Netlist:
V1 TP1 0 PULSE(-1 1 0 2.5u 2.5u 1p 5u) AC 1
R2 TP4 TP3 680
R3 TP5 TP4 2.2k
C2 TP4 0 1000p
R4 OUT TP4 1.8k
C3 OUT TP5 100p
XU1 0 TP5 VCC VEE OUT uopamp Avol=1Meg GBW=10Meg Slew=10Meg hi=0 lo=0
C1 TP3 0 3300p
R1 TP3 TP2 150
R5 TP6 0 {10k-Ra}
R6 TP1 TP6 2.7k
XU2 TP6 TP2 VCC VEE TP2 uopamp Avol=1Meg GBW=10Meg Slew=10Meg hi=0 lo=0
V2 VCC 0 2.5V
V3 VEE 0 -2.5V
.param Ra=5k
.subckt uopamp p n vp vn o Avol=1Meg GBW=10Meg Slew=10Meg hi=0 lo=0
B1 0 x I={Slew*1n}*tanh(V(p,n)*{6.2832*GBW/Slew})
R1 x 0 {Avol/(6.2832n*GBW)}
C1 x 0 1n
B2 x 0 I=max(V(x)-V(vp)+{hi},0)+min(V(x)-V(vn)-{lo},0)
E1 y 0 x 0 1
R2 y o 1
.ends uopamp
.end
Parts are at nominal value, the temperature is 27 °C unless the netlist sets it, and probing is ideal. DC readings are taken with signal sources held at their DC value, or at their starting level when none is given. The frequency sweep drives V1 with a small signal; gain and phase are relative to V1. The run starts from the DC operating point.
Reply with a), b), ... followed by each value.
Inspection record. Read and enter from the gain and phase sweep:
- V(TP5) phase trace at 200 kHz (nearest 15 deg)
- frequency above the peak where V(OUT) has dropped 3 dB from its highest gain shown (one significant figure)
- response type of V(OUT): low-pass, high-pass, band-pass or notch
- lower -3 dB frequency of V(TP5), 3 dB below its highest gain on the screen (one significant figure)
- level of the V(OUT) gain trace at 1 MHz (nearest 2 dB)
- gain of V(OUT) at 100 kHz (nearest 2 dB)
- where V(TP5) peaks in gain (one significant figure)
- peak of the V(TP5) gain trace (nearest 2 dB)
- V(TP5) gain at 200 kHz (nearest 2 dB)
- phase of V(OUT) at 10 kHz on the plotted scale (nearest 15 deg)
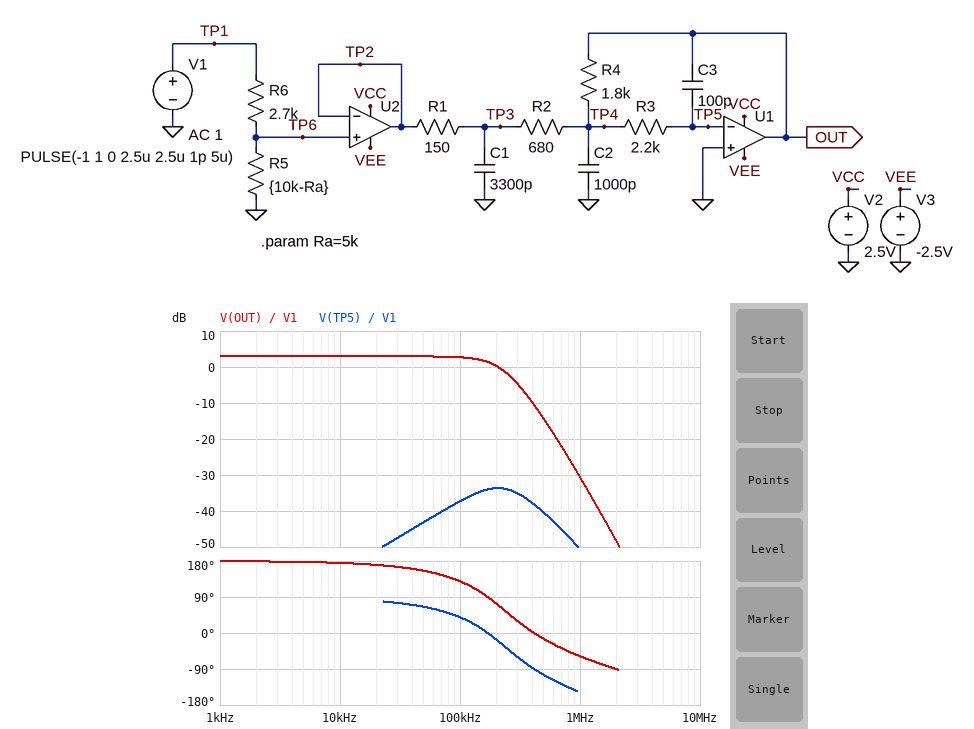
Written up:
a) -15 deg
b) 200 kHz
c) low-pass
d) 100 kHz
e) -30 dB
f) 2 dB
g) 200 kHz
h) -34 dB
i) -34 dB
j) 180 deg
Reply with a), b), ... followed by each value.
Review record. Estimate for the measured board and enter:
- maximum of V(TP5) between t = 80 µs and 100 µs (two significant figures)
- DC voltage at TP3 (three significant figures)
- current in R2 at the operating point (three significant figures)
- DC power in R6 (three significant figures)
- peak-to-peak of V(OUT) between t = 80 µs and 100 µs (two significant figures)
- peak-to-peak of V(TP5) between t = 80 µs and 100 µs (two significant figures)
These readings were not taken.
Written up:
a) 17 mV
b) -532 mV
c) 782 µA
d) 45.5 µW
e) 1.7 V
f) 35 mV
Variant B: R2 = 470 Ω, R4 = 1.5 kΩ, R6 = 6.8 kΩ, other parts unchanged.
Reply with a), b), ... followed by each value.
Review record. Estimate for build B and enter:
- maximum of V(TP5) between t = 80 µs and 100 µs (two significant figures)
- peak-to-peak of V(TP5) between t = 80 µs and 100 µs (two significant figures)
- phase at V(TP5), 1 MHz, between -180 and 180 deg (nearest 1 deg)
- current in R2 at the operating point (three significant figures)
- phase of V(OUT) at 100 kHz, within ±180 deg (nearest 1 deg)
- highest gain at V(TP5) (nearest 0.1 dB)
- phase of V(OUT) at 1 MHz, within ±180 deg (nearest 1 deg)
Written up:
a) 12 mV
b) 24 mV
c) -141 deg
d) 683 µA
e) 130 deg
f) -36.7 dB
g) -51 deg
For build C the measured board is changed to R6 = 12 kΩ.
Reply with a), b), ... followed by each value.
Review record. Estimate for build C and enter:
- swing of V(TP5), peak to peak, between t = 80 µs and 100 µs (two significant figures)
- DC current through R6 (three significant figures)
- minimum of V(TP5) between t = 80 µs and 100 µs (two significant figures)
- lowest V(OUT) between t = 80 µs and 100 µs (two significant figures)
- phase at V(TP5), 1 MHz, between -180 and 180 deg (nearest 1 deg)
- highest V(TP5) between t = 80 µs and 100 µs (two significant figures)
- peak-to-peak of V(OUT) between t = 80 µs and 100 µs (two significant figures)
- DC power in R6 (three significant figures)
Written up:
a) 16 mV
b) 58.8 µA
c) -7.8 mV
d) -380 mV
e) -148 deg
f) 7.8 mV
g) 760 mV
h) 41.5 µW
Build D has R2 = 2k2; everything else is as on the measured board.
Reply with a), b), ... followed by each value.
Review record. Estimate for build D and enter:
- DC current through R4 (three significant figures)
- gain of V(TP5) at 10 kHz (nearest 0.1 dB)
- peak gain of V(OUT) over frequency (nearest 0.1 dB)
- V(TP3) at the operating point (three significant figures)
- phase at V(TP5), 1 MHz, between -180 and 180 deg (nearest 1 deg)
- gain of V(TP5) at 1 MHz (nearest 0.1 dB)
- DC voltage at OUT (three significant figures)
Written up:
a) 276 µA
b) -66.1 dB
c) -5.1 dB
d) -608 mV
e) -159 deg
f) -60.1 dB
g) 497 mV
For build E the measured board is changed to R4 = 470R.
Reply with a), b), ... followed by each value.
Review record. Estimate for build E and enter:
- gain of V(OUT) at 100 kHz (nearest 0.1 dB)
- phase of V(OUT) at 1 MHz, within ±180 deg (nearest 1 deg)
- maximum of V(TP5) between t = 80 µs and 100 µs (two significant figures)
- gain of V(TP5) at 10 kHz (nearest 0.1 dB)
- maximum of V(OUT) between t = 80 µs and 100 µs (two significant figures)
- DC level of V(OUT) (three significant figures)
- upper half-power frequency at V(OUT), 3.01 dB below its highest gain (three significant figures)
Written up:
a) -8.8 dB
b) -42 deg
c) 5.0 mV
d) -68.7 dB
e) 290 mV
f) 368 mV
g) 368 kHz
